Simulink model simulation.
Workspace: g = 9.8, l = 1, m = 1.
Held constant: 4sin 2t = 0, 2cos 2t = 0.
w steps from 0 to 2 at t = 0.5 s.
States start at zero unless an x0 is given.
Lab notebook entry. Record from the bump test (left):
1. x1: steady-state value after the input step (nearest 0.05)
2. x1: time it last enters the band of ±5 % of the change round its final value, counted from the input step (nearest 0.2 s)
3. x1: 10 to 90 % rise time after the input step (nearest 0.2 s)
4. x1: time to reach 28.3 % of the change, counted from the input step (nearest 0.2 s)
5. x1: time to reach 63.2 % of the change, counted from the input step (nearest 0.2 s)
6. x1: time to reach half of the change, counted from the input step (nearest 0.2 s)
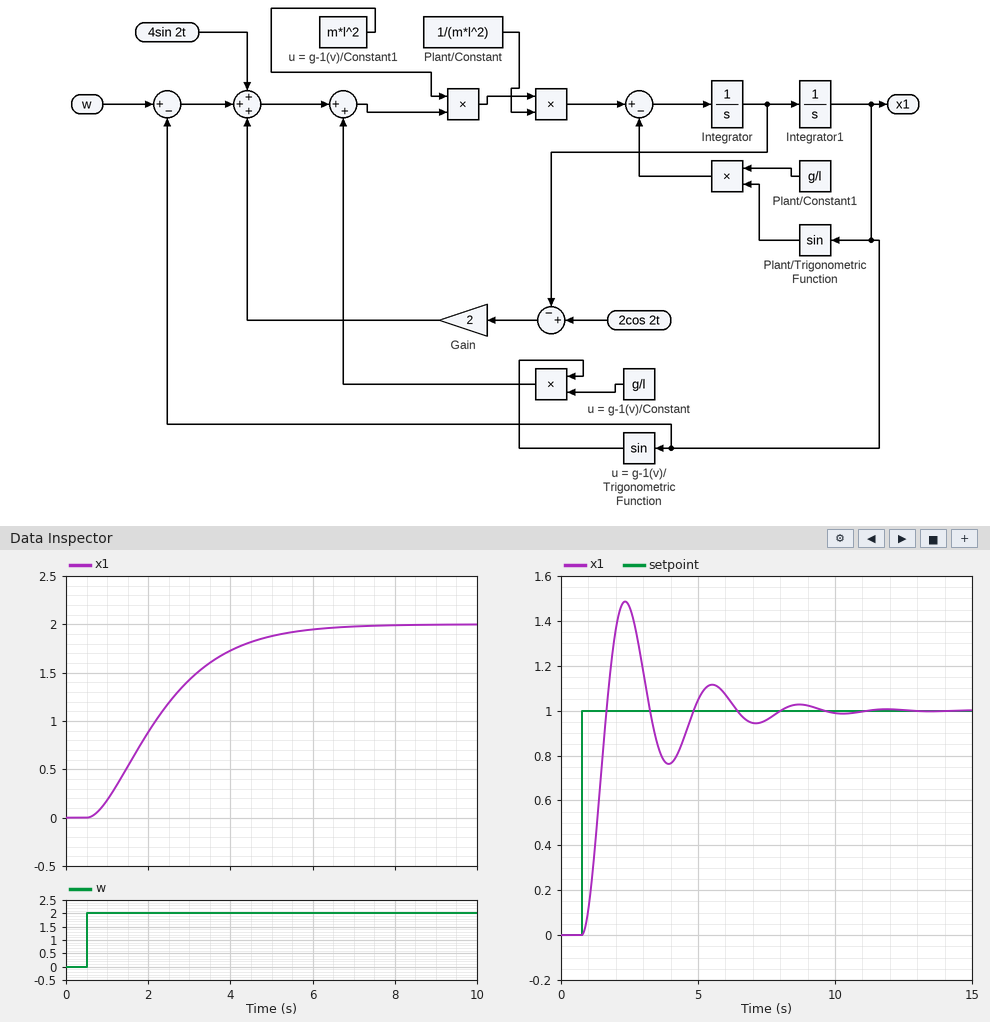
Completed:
2.00
4.8 s
3.4 s
1.0 s
2.2 s
1.6 s
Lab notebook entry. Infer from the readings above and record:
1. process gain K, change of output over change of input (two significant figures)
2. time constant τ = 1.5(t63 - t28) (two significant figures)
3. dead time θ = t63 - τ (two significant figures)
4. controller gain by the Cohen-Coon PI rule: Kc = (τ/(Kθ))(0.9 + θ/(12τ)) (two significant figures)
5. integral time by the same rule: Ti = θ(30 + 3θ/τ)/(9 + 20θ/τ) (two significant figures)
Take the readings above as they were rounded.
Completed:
1.0
1.8 s
0.40 s
4.1
0.91 s
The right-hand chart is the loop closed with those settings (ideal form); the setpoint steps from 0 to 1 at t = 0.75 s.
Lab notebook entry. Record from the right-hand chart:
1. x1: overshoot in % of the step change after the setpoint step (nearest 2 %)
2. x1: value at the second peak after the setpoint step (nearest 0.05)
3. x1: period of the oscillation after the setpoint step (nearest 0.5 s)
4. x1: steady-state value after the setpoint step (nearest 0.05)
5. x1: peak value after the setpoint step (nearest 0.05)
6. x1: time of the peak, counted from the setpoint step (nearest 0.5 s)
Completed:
48 %
1.10
3.0 s
1.00
1.50
1.5 s
